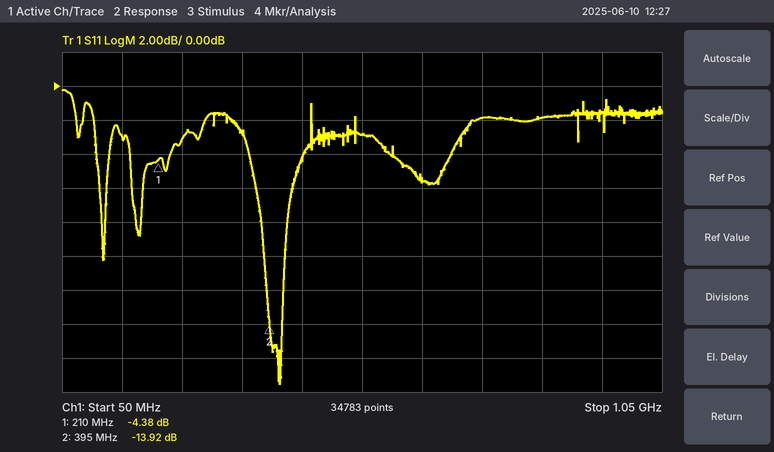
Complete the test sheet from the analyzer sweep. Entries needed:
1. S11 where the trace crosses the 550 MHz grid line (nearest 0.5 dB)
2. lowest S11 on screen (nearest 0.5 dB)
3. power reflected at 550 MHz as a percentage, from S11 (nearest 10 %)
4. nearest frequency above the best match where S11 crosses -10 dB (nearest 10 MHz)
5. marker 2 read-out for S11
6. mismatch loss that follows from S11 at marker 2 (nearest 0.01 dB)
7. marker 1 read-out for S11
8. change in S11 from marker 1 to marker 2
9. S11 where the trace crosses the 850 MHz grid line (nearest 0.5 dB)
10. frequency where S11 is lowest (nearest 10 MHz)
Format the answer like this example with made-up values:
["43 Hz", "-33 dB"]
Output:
["-3.0 dB", "-17.5 dB", "50 %", "420 MHz", "-13.92 dB", "0.18 dB", "-4.38 dB", "-9.54 dB", "-2.0 dB", "410 MHz"]
